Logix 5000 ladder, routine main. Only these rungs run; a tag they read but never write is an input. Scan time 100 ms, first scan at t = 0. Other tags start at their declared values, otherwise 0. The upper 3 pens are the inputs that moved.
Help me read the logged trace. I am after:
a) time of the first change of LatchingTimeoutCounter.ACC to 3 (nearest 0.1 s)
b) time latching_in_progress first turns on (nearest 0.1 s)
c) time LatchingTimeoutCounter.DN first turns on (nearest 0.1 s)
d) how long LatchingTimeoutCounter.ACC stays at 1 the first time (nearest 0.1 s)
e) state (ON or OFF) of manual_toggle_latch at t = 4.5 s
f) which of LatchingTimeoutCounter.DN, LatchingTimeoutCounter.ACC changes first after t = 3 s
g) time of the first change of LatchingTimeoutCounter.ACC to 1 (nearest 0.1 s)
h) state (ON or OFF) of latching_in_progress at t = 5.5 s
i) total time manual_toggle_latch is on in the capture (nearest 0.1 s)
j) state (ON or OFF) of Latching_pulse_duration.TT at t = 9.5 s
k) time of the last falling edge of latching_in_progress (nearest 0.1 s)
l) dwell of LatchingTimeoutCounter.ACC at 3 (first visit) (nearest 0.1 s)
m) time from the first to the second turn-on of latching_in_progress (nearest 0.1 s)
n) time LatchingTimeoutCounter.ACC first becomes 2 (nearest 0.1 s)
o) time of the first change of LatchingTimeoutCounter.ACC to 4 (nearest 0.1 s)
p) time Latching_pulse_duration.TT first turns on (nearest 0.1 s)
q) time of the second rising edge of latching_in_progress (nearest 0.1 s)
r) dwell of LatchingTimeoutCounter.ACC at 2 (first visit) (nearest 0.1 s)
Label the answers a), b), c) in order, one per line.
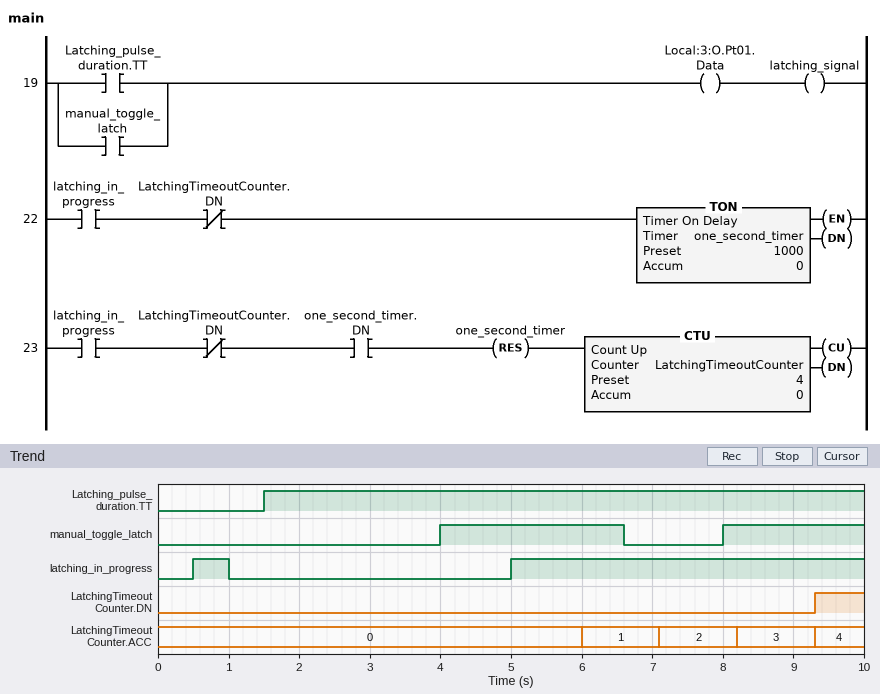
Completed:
a) 8.2 s
b) 0.5 s
c) 9.3 s
d) 1.1 s
e) ON
f) LatchingTimeoutCounter.ACC
g) 6.0 s
h) ON
i) 4.6 s
j) ON
k) 1.0 s
l) 1.1 s
m) 4.5 s
n) 7.1 s
o) 9.3 s
p) 1.5 s
q) 5.0 s
r) 1.1 s
